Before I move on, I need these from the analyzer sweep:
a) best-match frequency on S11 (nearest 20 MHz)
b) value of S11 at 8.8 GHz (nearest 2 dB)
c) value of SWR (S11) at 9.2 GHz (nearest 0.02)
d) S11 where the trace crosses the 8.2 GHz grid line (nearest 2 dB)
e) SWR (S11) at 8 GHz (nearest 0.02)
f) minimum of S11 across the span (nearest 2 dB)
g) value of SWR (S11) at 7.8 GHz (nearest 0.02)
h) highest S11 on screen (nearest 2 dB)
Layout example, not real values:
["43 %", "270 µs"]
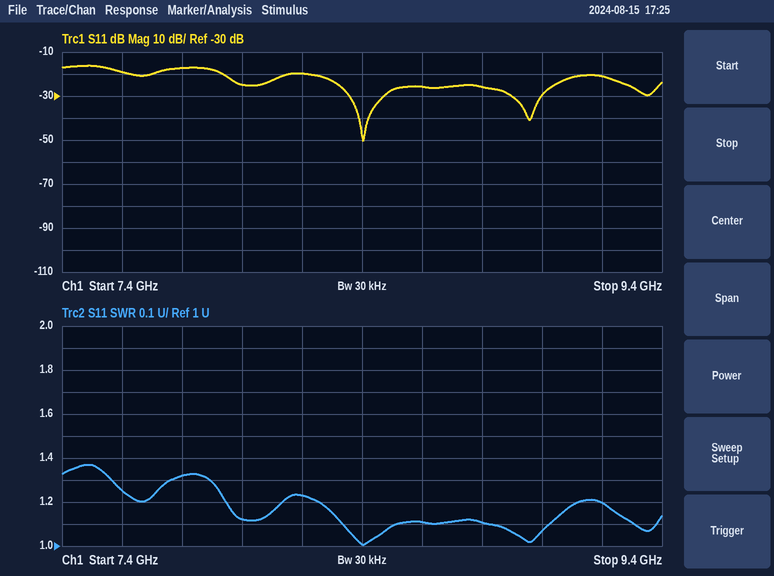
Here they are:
["8.40 GHz", "-26 dB", "1.20", "-20 dB", "1.12", "-50 dB", "1.32", "-16 dB"]
